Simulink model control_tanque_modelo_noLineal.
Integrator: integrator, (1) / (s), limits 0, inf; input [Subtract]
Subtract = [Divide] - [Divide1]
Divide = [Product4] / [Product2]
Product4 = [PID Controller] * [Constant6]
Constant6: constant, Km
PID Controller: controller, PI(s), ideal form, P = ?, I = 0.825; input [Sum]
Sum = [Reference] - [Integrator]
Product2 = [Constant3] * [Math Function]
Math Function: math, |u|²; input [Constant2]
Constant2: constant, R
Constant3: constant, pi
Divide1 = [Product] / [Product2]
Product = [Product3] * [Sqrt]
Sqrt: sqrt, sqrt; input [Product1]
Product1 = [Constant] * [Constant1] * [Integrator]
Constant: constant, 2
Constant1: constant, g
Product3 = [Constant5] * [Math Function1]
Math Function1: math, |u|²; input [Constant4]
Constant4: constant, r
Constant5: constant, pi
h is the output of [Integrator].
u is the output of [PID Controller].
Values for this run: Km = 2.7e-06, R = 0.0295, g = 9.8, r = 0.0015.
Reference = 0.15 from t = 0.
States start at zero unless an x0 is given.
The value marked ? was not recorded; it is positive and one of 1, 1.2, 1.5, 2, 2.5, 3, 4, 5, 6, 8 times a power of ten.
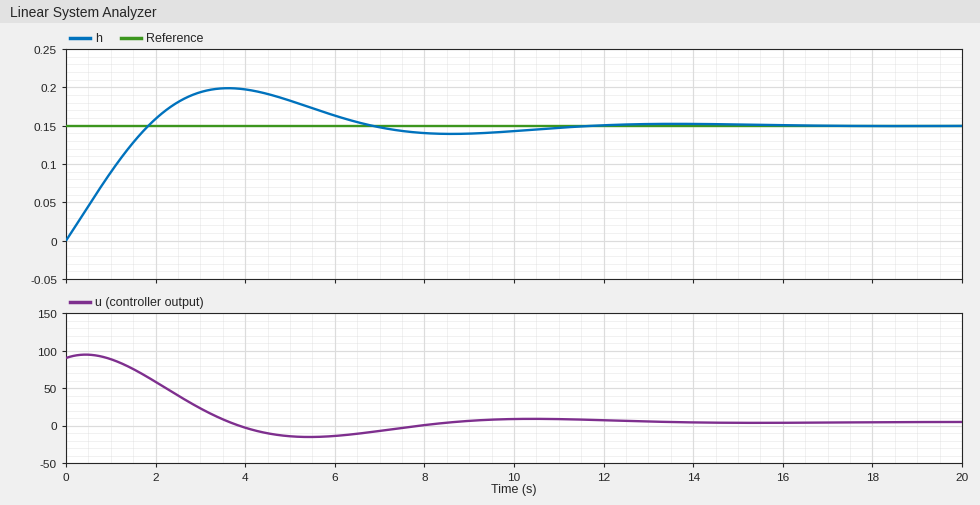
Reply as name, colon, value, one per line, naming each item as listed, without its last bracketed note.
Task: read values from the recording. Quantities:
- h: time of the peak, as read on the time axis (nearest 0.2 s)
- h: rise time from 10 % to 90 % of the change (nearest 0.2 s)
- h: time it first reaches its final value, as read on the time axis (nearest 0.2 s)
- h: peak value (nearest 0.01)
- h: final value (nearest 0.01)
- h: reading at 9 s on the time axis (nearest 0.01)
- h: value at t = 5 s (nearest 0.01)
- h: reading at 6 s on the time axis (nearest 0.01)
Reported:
h: time of the peak, as read on the time axis: 3.6 s
h: rise time from 10 % to 90 % of the change: 1.4 s
h: time it first reaches its final value, as read on the time axis: 1.8 s
h: peak value: 0.20
h: final value: 0.15
h: reading at 9 s on the time axis: 0.14
h: value at t = 5 s: 0.18
h: reading at 6 s on the time axis: 0.16
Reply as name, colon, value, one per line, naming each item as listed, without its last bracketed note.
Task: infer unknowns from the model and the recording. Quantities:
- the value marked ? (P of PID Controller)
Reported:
the value marked ?: 600
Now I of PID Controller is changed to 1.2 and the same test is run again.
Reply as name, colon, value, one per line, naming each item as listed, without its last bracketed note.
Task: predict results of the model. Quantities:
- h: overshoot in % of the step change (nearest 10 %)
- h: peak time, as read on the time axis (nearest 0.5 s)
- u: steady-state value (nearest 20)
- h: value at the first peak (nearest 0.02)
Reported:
h: overshoot in % of the step change: 40 %
h: peak time, as read on the time axis: 3.0 s
u: steady-state value: 0
h: value at the first peak: 0.20
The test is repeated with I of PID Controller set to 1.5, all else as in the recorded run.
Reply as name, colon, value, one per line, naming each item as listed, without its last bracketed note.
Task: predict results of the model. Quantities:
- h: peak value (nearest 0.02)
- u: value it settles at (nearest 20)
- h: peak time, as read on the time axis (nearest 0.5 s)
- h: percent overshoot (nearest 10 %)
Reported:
h: peak value: 0.22
u: value it settles at: 0
h: peak time, as read on the time axis: 3.0 s
h: percent overshoot: 40 %
